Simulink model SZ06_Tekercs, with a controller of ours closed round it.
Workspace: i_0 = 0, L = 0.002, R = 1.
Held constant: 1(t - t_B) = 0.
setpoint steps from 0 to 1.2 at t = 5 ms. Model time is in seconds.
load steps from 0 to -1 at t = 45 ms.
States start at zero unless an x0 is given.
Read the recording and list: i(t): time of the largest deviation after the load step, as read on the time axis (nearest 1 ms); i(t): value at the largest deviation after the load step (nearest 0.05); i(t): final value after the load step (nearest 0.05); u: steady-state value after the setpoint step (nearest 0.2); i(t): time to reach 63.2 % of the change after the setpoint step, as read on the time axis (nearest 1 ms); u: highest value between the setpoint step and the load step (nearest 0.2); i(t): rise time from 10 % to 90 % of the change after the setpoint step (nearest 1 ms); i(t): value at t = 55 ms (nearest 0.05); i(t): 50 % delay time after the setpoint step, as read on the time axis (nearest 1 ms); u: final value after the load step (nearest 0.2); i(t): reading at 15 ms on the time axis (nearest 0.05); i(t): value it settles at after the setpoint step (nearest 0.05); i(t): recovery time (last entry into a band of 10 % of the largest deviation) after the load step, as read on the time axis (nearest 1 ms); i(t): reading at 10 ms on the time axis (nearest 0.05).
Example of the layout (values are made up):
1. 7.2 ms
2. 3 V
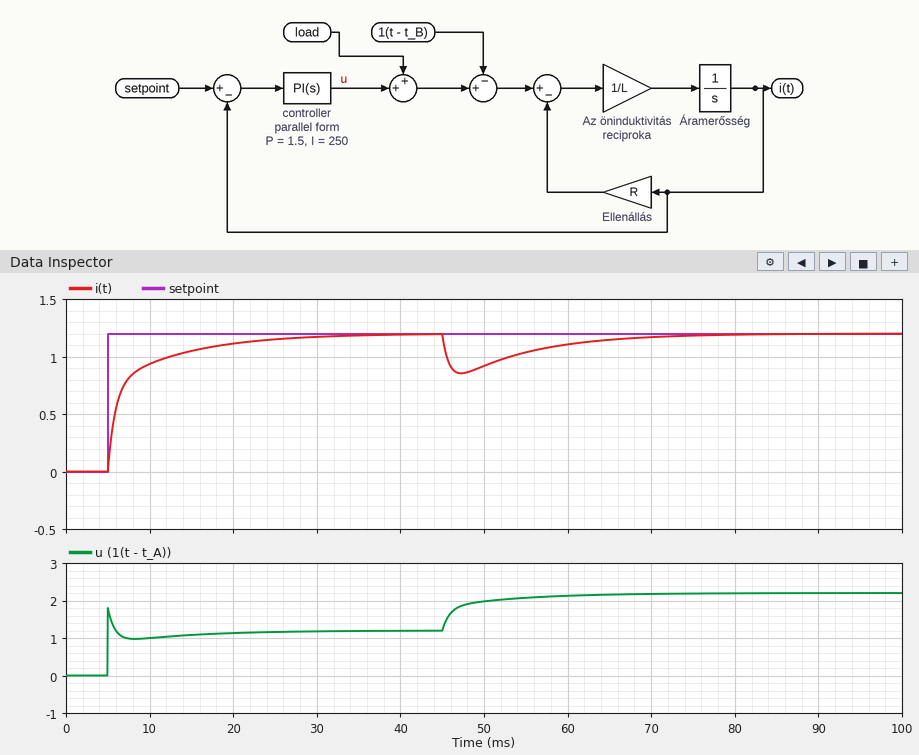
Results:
1. 47 ms
2. 0.85
3. 1.20
4. 1.2
5. 7 ms
6. 1.8
7. 12 ms
8. 1.05
9. 6 ms
10. 2.2
11. 1.05
12. 1.20
13. 69 ms
14. 0.95
